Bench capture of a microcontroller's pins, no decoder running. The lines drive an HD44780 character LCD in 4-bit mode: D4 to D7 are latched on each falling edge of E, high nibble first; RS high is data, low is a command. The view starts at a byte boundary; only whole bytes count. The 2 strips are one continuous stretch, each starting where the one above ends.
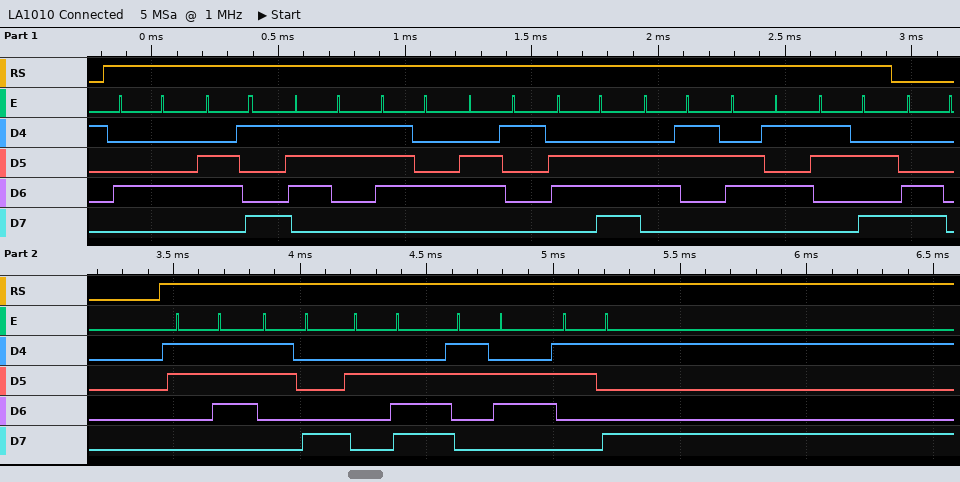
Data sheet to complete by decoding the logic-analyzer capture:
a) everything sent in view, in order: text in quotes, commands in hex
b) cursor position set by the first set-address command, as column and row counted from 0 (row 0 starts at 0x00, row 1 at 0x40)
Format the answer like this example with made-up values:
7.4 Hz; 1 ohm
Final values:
"Distance:" 0xC0 "78.69"; column 0, row 1
